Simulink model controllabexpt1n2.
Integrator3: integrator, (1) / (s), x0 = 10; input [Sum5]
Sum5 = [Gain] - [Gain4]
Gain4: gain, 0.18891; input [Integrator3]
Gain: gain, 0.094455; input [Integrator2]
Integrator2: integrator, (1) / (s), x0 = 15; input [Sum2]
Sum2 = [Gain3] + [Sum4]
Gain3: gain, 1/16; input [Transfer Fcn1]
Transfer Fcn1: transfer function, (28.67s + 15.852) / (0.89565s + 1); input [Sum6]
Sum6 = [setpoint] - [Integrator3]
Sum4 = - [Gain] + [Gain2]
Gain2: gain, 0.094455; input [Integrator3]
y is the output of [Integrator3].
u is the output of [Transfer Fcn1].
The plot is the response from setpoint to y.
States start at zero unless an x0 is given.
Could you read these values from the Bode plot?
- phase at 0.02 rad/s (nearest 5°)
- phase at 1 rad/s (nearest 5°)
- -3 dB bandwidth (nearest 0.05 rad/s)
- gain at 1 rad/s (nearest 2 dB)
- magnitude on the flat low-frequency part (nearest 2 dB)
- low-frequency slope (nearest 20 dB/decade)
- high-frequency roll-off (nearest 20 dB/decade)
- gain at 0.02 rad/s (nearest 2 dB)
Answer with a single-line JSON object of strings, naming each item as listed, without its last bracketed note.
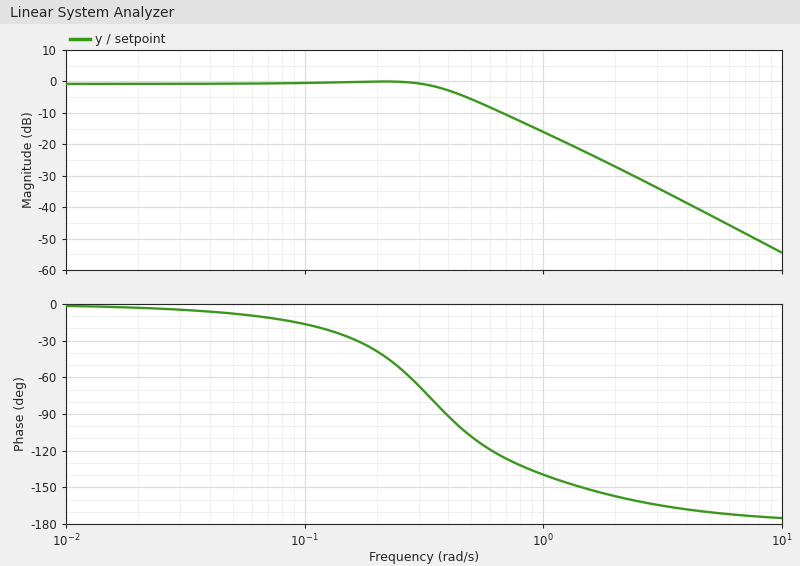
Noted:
{"phase at 0.02 rad/s": "-5°", "phase at 1 rad/s": "-140°", "-3 dB bandwidth": "0.45 rad/s", "gain at 1 rad/s": "-16 dB", "magnitude on the flat low-frequency part": "0 dB", "low-frequency slope": "0 dB/decade", "high-frequency roll-off": "-40 dB/decade", "gain at 0.02 rad/s": "0 dB"}
